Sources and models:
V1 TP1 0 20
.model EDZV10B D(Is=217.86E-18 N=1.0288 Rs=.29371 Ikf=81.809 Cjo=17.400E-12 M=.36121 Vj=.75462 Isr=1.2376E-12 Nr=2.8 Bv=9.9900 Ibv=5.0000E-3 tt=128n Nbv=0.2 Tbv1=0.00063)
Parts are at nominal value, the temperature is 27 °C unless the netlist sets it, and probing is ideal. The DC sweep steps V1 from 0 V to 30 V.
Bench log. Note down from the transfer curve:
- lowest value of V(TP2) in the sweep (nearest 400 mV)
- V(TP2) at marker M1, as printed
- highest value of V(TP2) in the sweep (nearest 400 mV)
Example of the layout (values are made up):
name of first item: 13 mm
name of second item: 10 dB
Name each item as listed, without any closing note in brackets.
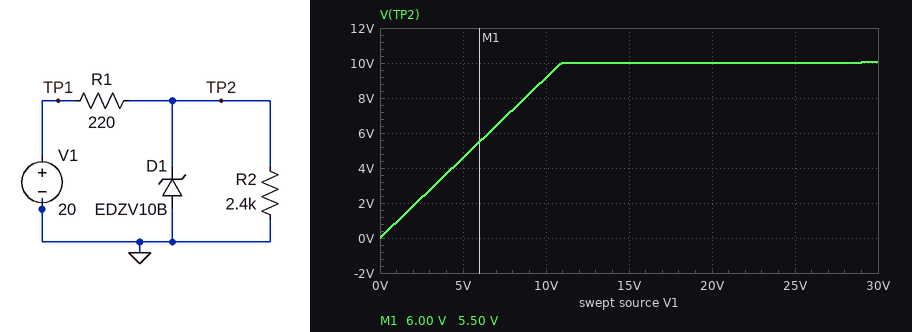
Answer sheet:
lowest value of V(TP2) in the sweep: 0 V
V(TP2) at marker M1, as printed: 5.50 V
highest value of V(TP2) in the sweep: 10.0 V
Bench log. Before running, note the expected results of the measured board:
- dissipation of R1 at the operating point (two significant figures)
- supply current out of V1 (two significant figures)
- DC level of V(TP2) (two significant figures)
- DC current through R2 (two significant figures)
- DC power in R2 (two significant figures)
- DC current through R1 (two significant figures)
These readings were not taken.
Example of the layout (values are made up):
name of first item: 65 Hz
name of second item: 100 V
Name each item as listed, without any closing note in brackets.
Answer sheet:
dissipation of R1 at the operating point: 450 mW
supply current out of V1: 45 mA
DC level of V(TP2): 10 V
DC current through R2: 4.2 mA
DC power in R2: 42 mW
DC current through R1: 45 mA
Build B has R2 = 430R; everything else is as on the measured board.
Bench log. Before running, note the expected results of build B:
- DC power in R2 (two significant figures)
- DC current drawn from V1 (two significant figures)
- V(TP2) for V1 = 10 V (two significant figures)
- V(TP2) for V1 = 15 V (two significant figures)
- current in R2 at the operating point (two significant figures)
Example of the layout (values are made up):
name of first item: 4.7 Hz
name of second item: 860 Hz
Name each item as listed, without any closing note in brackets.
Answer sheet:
DC power in R2: 230 mW
DC current drawn from V1: 45 mA
V(TP2) for V1 = 10 V: 6.6 V
V(TP2) for V1 = 15 V: 9.9 V
current in R2 at the operating point: 23 mA
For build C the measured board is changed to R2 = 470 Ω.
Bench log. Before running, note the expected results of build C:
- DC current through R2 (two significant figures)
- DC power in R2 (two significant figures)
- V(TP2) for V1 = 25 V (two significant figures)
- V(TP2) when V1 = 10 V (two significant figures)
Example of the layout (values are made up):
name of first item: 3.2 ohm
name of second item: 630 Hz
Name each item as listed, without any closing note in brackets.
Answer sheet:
DC current through R2: 21 mA
DC power in R2: 210 mW
V(TP2) for V1 = 25 V: 10 V
V(TP2) when V1 = 10 V: 6.8 V
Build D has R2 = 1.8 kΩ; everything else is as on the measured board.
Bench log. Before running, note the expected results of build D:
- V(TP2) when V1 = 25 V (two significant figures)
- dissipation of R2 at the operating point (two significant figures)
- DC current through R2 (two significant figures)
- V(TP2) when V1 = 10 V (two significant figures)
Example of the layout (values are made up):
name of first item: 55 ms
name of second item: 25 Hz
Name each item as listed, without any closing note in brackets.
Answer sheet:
V(TP2) when V1 = 25 V: 10 V
dissipation of R2 at the operating point: 56 mW
DC current through R2: 5.6 mA
V(TP2) when V1 = 10 V: 8.9 V
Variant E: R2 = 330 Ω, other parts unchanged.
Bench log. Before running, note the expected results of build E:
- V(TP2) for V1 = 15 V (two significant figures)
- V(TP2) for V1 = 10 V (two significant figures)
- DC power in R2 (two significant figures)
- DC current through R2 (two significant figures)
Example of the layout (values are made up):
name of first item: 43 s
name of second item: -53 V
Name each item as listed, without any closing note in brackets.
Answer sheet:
V(TP2) for V1 = 15 V: 9.0 V
V(TP2) for V1 = 10 V: 6.0 V
DC power in R2: 300 mW
DC current through R2: 30 mA
